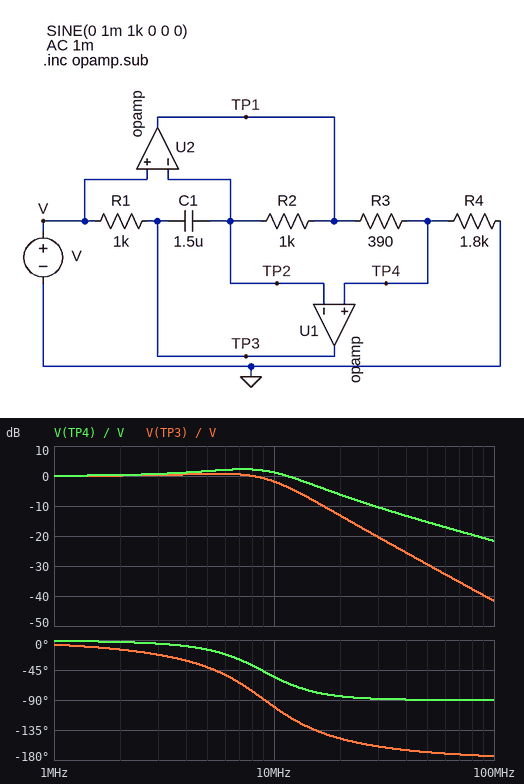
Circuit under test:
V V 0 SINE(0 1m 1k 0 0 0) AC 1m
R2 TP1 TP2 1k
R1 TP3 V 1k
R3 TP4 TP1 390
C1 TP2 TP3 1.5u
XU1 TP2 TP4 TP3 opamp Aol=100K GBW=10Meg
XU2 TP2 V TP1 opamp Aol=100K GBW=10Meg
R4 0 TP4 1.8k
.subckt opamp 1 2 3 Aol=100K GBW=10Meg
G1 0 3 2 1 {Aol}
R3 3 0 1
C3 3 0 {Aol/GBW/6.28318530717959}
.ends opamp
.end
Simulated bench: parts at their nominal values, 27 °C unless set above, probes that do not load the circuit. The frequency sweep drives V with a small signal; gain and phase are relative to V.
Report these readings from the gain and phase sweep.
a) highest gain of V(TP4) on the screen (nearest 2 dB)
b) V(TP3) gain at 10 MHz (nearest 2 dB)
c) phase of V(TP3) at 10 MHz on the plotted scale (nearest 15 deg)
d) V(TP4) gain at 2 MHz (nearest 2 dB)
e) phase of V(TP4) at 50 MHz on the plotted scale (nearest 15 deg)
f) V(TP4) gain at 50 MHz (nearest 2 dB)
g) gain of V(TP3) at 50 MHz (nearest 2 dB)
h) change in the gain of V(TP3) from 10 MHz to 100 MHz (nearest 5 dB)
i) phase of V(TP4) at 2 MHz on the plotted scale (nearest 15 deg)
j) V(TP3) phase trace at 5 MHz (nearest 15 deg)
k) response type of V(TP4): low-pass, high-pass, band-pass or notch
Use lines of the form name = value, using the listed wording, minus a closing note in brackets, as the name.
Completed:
highest gain of V(TP4) on the screen = 2 dB
V(TP3) gain at 10 MHz = -2 dB
phase of V(TP3) at 10 MHz on the plotted scale = -105 deg
V(TP4) gain at 2 MHz = 0 dB
phase of V(TP4) at 50 MHz on the plotted scale = -90 deg
V(TP4) gain at 50 MHz = -16 dB
gain of V(TP3) at 50 MHz = -30 dB
change in the gain of V(TP3) from 10 MHz to 100 MHz = -40 dB
phase of V(TP4) at 2 MHz on the plotted scale = 0 deg
V(TP3) phase trace at 5 MHz = -45 deg
response type of V(TP4): low-pass, high-pass, band-pass or notch = low-pass
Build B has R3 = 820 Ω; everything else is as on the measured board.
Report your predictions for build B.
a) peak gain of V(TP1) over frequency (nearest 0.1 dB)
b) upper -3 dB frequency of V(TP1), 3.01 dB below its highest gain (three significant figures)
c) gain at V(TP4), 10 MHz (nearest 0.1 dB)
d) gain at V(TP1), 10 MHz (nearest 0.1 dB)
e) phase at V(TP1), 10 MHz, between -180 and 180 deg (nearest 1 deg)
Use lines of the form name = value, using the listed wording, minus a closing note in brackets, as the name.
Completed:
peak gain of V(TP1) over frequency = 4.6 dB
upper -3 dB frequency of V(TP1), 3.01 dB below its highest gain = 11.1 MHz
gain at V(TP4), 10 MHz = -0.7 dB
gain at V(TP1), 10 MHz = 2.6 dB
phase at V(TP1), 10 MHz, between -180 and 180 deg = -62 deg
